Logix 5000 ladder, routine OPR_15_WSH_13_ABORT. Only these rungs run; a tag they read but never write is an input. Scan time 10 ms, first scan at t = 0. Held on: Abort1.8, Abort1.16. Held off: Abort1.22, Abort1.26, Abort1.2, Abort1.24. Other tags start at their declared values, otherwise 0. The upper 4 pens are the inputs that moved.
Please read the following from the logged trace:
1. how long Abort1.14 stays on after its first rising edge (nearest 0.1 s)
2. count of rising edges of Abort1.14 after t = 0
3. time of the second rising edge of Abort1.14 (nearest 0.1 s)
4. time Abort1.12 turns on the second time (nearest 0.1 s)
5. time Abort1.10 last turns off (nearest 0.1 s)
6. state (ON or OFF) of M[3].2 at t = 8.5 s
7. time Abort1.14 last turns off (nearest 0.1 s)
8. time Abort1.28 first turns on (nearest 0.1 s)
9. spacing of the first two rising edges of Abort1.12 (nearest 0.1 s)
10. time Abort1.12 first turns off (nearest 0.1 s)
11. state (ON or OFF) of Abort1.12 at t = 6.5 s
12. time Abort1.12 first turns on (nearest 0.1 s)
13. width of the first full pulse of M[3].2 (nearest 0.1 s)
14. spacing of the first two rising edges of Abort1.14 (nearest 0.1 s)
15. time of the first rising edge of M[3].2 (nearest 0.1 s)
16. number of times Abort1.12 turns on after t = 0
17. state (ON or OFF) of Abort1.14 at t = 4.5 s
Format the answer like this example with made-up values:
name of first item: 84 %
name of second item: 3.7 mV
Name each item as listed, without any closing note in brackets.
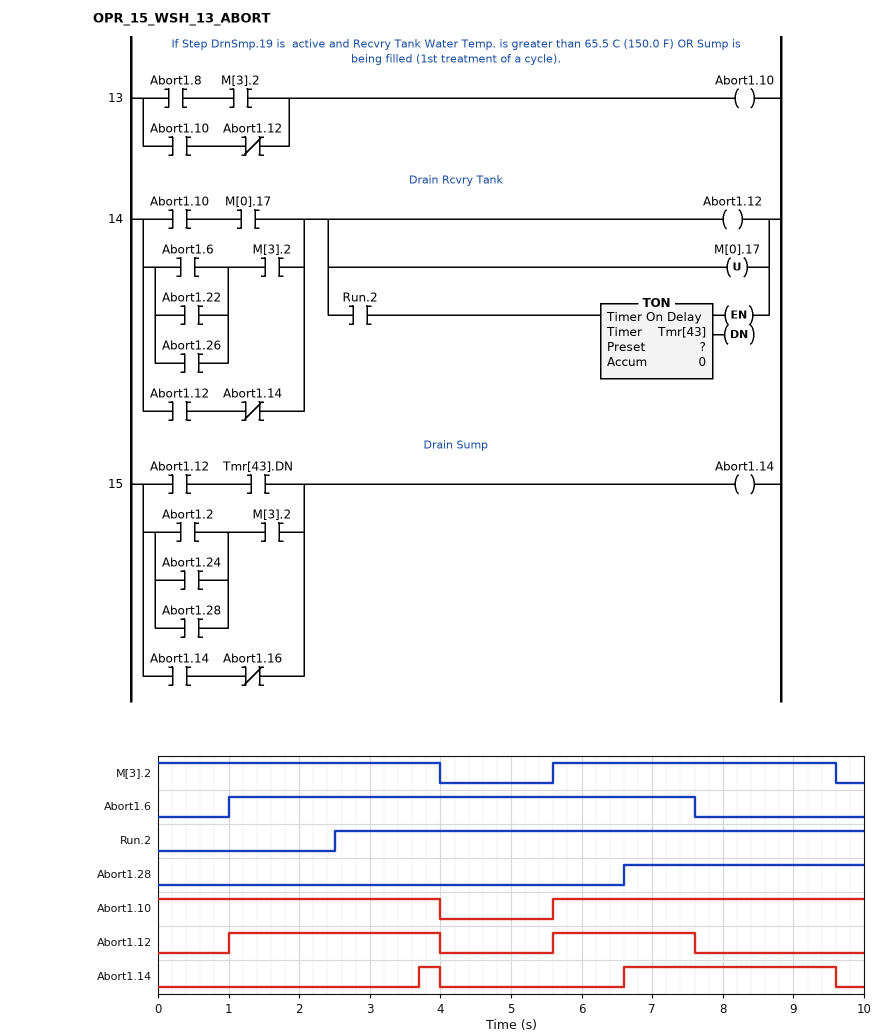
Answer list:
how long Abort1.14 stays on after its first rising edge: 0.3 s
count of rising edges of Abort1.14 after t = 0: 2
time of the second rising edge of Abort1.14: 6.6 s
time Abort1.12 turns on the second time: 5.6 s
time Abort1.10 last turns off: 4.0 s
state (ON or OFF) of M[3].2 at t = 8.5 s: ON
time Abort1.14 last turns off: 9.6 s
time Abort1.28 first turns on: 6.6 s
spacing of the first two rising edges of Abort1.12: 4.6 s
time Abort1.12 first turns off: 4.0 s
state (ON or OFF) of Abort1.12 at t = 6.5 s: ON
time Abort1.12 first turns on: 1.0 s
width of the first full pulse of M[3].2: 4.0 s
spacing of the first two rising edges of Abort1.14: 2.9 s
time of the first rising edge of M[3].2: 5.6 s
number of times Abort1.12 turns on after t = 0: 2
state (ON or OFF) of Abort1.14 at t = 4.5 s: OFF
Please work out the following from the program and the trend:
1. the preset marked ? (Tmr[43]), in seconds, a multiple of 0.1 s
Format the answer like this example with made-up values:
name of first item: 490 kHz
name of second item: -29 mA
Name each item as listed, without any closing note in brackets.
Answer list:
the preset marked ? (Tmr[43]), in seconds, a multiple of 0.1 s: 1.2 s
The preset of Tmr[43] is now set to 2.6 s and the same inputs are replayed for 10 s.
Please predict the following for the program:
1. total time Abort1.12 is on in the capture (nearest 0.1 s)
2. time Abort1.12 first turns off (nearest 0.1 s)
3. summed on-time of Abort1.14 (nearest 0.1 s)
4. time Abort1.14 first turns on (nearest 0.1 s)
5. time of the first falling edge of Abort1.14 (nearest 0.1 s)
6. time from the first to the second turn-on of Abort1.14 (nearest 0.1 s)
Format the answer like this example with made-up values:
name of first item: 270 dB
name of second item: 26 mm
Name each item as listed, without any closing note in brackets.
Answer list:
total time Abort1.12 is on in the capture: 6.1 s
time Abort1.12 first turns off: 5.1 s
summed on-time of Abort1.14: 3.0 s
time Abort1.14 first turns on: 5.1 s
time of the first falling edge of Abort1.14: 5.1 s
time from the first to the second turn-on of Abort1.14: 1.5 s
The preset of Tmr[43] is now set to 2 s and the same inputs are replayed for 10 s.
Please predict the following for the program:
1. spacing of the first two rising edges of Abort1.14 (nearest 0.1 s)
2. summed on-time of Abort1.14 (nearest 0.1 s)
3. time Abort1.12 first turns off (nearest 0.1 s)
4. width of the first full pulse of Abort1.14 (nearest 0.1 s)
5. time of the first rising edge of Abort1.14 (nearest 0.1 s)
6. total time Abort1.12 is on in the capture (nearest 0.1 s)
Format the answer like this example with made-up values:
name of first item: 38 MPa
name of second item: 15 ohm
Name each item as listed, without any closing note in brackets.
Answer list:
spacing of the first two rising edges of Abort1.14: 2.1 s
summed on-time of Abort1.14: 3.0 s
time Abort1.12 first turns off: 4.5 s
width of the first full pulse of Abort1.14: 0.0 s
time of the first rising edge of Abort1.14: 4.5 s
total time Abort1.12 is on in the capture: 5.5 s
